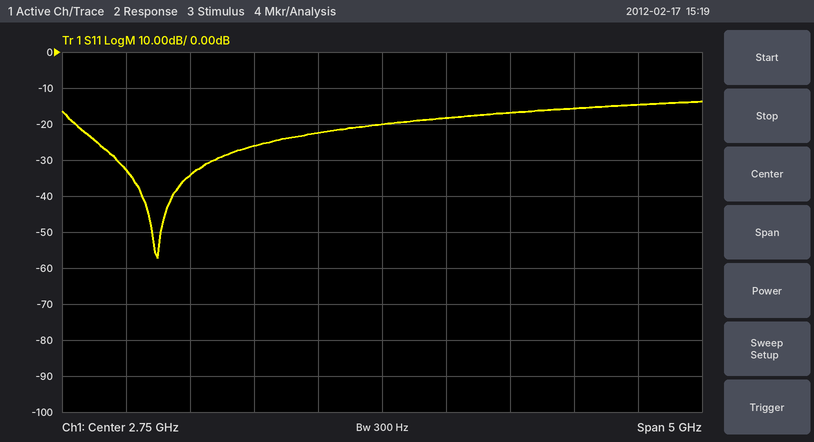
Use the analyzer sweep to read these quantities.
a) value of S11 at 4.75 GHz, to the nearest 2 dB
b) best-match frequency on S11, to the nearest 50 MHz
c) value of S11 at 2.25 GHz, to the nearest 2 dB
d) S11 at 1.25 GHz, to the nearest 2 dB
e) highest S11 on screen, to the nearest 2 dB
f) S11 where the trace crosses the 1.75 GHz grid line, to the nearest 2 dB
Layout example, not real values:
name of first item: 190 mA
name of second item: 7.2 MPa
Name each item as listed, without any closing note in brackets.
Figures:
value of S11 at 4.75 GHz, to the nearest 2 dB: -14 dB
best-match frequency on S11, to the nearest 50 MHz: 1.00 GHz
value of S11 at 2.25 GHz, to the nearest 2 dB: -22 dB
S11 at 1.25 GHz, to the nearest 2 dB: -34 dB
highest S11 on screen, to the nearest 2 dB: -14 dB
S11 where the trace crosses the 1.75 GHz grid line, to the nearest 2 dB: -26 dB
